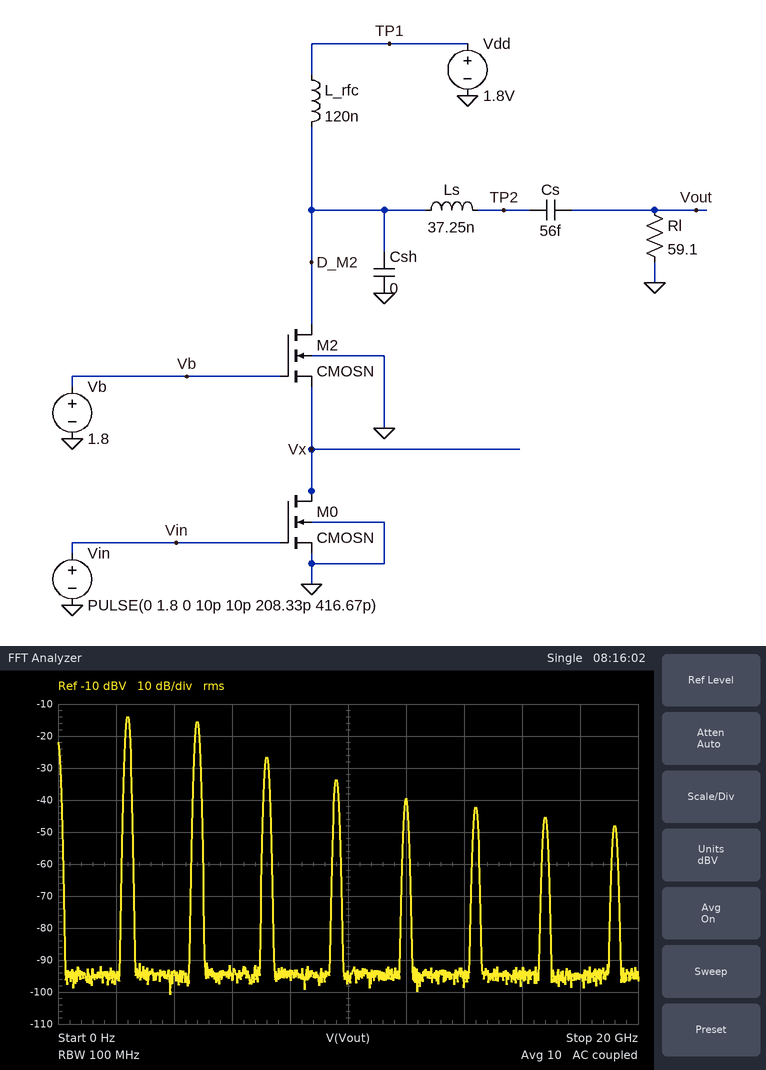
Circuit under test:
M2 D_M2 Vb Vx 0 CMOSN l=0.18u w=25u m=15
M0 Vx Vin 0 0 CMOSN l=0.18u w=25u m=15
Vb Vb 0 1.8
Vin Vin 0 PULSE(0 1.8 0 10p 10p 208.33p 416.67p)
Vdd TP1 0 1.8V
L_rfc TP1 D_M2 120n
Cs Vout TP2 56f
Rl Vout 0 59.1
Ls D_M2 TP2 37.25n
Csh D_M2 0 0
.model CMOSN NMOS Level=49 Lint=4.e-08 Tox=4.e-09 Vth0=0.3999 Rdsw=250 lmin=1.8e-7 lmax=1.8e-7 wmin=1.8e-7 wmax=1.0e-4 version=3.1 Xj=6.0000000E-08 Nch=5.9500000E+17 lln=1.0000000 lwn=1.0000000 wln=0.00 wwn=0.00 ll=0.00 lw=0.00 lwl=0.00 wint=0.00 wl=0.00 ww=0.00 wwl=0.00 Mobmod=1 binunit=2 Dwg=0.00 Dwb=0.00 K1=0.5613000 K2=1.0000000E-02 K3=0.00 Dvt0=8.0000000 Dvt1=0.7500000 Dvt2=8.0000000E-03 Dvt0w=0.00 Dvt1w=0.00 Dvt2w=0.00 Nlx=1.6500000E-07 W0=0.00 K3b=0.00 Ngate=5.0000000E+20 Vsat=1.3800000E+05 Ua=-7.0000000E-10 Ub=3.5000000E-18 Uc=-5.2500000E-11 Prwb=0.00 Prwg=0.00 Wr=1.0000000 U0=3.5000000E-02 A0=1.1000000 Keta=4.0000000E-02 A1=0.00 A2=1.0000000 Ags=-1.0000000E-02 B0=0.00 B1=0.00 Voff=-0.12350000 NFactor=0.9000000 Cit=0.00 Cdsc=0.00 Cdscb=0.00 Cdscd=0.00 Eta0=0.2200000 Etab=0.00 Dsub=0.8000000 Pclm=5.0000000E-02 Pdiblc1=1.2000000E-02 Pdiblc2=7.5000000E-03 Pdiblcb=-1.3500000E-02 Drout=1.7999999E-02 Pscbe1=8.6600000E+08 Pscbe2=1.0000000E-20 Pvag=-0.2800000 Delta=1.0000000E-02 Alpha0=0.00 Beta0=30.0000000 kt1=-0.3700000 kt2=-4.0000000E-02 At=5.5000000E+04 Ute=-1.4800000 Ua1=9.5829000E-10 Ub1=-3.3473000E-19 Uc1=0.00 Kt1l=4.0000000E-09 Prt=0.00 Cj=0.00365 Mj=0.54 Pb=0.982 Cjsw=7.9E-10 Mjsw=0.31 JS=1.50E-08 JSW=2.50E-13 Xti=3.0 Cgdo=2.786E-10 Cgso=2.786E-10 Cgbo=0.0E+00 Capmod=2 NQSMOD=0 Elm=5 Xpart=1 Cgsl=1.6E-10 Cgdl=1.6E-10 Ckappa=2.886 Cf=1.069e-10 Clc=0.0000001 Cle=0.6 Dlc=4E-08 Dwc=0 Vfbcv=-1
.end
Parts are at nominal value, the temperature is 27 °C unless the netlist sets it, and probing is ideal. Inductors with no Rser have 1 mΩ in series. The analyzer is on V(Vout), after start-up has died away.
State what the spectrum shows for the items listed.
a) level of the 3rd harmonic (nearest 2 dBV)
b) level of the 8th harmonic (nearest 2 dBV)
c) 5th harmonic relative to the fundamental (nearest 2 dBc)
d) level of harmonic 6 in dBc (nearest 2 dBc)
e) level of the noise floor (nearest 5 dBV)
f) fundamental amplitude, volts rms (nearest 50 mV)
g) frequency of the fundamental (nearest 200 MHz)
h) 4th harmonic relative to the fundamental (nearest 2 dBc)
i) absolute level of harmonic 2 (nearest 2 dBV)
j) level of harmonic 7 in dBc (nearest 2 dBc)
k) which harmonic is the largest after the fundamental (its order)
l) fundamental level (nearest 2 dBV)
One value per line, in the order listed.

-26 dBV
-48 dBV
-26 dBc
-28 dBc
-95 dBV
200 mV
2.4 GHz
-20 dBc
-16 dBV
-32 dBc
2
-14 dBV
